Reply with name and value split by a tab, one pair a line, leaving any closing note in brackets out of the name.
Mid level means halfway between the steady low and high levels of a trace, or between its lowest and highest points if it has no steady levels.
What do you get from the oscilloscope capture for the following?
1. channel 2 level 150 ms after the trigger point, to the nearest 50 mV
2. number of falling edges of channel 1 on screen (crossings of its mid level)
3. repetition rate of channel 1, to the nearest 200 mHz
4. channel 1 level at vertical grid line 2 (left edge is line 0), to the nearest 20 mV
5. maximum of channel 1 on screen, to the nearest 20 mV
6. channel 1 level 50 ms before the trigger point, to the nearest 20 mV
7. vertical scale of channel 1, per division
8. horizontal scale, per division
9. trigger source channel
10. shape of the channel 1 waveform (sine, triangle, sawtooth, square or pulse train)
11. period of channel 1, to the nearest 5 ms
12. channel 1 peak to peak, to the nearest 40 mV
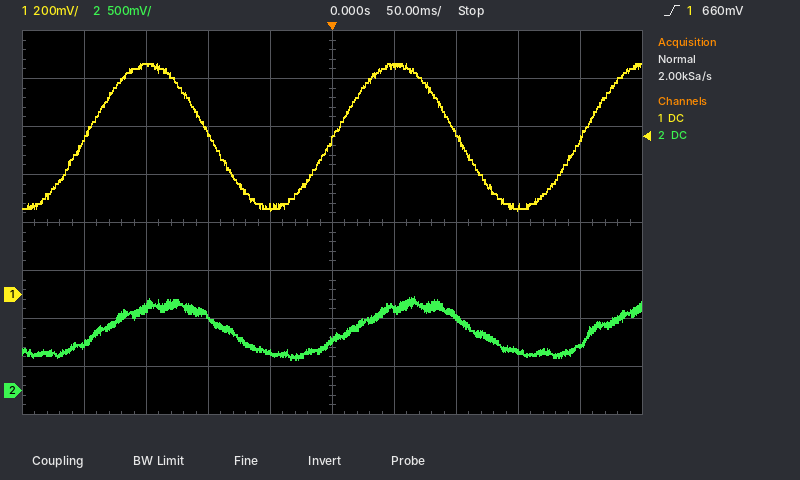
channel 2 level 150 ms after the trigger point, to the nearest 50 mV	400 mV
number of falling edges of channel 1 on screen	2
repetition rate of channel 1, to the nearest 200 mHz	5.0 Hz
channel 1 level at vertical grid line 2 (left edge is line 0), to the nearest 20 mV	960 mV
maximum of channel 1 on screen, to the nearest 20 mV	960 mV
channel 1 level 50 ms before the trigger point, to the nearest 20 mV	360 mV
vertical scale of channel 1, per division	200 mV
horizontal scale, per division	50 ms
trigger source channel	channel 1
shape of the channel 1 waveform	sine
period of channel 1, to the nearest 5 ms	200 ms
channel 1 peak to peak, to the nearest 40 mV	600 mV
